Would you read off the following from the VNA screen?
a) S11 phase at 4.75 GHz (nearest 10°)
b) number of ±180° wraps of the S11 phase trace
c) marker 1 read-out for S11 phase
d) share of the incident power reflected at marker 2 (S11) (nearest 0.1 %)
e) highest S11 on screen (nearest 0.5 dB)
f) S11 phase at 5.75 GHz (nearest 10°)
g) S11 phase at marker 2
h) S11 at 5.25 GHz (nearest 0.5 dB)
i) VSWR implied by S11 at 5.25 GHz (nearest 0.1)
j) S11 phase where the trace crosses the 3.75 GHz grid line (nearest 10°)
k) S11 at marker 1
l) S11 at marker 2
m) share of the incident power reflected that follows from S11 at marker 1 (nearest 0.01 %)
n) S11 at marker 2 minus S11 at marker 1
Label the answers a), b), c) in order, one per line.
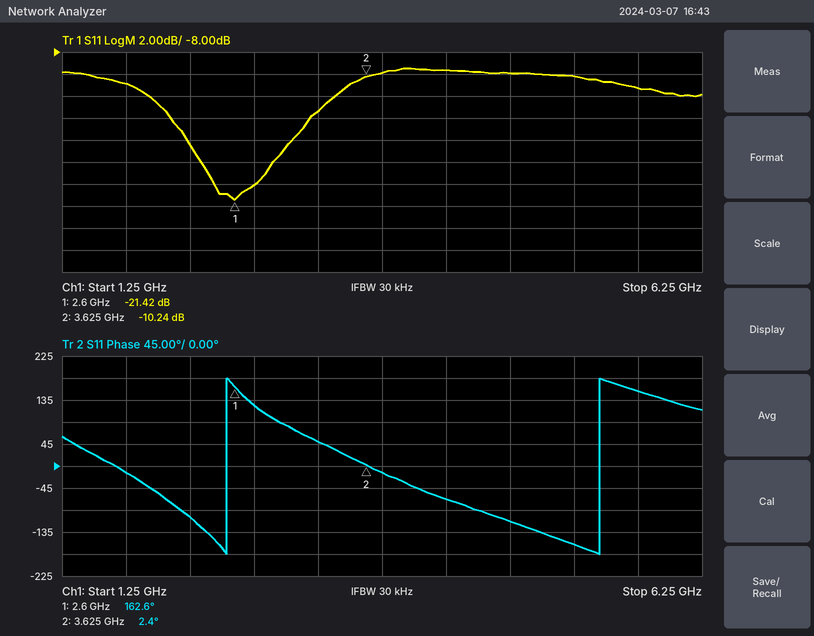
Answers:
a) -110°
b) 2
c) 162.6°
d) 9.5 %
e) -9.5 dB
f) 150°
g) 2.4°
h) -10.0 dB
i) 1.9
j) -10°
k) -21.42 dB
l) -10.24 dB
m) 0.72 %
n) 11.18 dB
